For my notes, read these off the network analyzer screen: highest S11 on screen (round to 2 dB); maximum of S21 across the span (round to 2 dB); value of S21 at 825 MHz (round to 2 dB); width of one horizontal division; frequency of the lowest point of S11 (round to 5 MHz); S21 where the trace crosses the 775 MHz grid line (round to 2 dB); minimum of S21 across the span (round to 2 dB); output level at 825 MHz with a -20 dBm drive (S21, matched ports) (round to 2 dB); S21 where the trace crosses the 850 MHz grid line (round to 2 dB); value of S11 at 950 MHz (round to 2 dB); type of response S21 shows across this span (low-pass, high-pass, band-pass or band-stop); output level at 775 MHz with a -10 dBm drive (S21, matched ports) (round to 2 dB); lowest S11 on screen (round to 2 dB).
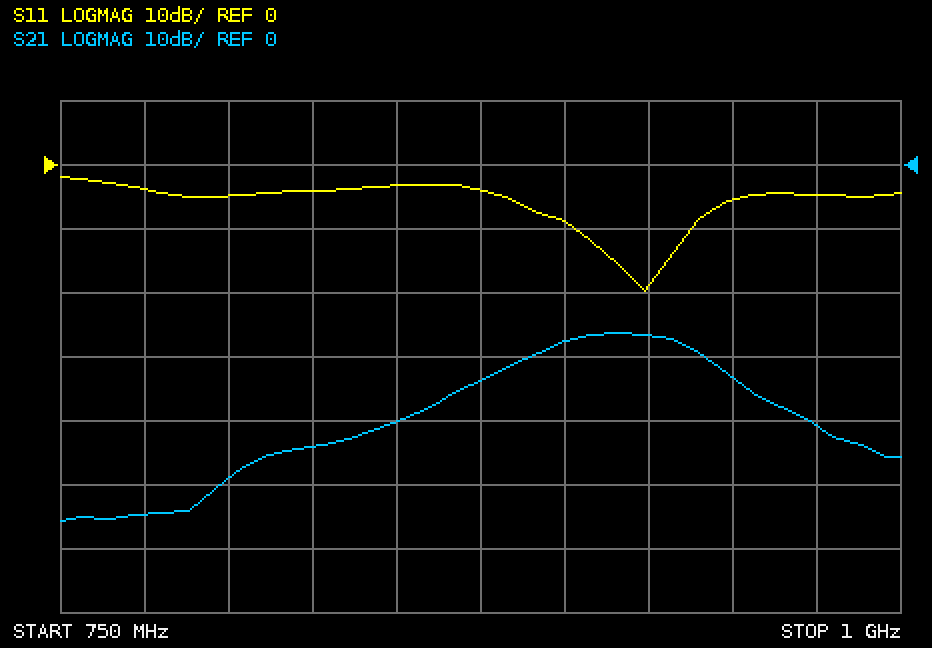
-2 dB
-26 dB
-44 dB
25 MHz
925 MHz
-54 dB
-56 dB
-64 dBm
-40 dB
-6 dB
band-pass
-64 dBm
-20 dB
